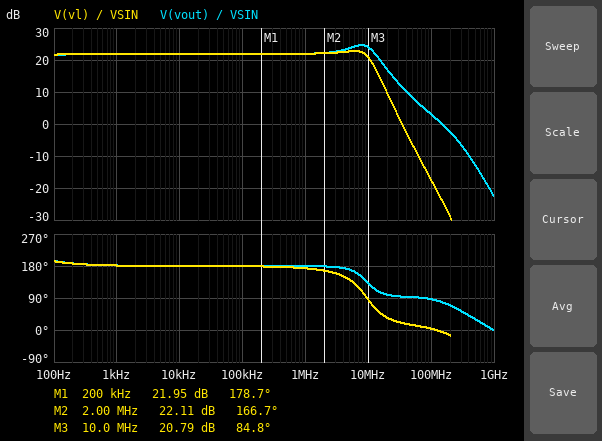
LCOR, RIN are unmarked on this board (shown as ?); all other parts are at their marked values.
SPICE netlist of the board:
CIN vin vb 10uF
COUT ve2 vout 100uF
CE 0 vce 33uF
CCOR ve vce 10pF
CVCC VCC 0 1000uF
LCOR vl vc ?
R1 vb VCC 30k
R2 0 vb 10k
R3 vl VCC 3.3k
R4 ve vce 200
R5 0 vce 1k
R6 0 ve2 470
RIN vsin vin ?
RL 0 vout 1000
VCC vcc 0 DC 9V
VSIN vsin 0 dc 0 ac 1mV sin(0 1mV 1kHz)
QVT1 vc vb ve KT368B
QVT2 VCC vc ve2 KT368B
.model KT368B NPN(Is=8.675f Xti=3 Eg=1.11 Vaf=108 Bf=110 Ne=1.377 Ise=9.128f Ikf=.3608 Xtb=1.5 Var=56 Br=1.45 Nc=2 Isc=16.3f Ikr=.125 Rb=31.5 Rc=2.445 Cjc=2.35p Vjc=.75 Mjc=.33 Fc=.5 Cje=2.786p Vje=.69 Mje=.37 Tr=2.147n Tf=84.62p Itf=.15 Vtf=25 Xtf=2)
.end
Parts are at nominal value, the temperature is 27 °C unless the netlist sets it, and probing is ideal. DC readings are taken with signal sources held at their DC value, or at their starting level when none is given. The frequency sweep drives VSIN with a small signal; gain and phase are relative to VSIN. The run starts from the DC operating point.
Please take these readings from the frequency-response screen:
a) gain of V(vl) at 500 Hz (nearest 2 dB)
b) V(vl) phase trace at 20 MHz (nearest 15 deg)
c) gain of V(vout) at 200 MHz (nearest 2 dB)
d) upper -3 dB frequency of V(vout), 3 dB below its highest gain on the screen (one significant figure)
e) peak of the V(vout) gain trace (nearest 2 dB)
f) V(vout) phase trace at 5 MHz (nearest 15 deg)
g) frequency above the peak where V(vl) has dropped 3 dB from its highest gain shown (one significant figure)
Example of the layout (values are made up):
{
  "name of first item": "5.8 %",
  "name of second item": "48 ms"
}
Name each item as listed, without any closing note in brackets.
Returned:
{
  "gain of V(vl) at 500 Hz": "22 dB",
  "V(vl) phase trace at 20 MHz": "30 deg",
  "gain of V(vout) at 200 MHz": "-2 dB",
  "upper -3 dB frequency of V(vout), 3 dB below its highest gain on the screen": "10 MHz",
  "peak of the V(vout) gain trace": "24 dB",
  "V(vout) phase trace at 5 MHz": "165 deg",
  "frequency above the peak where V(vl) has dropped 3 dB from its highest gain shown": "10 MHz"
}
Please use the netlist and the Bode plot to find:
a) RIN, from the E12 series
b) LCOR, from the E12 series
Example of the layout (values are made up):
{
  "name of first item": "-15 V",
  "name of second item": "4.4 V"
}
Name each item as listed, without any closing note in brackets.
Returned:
{
  "RIN, from the E12 series": "390 Ω",
  "LCOR, from the E12 series": "56 µH"
}
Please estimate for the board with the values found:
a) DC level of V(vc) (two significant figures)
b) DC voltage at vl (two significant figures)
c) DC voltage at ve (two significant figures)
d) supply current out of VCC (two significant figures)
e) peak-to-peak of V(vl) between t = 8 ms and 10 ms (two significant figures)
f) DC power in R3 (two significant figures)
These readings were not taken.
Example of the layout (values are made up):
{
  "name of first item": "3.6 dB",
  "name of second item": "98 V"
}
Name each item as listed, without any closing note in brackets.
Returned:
{
  "DC level of V(vc)": "4.7 V",
  "DC voltage at vl": "4.7 V",
  "DC voltage at ve": "1.5 V",
  "supply current out of VCC": "9.9 mA",
  "peak-to-peak of V(vl) between t = 8 ms and 10 ms": "25 mV",
  "DC power in R3": "5.7 mW"
}
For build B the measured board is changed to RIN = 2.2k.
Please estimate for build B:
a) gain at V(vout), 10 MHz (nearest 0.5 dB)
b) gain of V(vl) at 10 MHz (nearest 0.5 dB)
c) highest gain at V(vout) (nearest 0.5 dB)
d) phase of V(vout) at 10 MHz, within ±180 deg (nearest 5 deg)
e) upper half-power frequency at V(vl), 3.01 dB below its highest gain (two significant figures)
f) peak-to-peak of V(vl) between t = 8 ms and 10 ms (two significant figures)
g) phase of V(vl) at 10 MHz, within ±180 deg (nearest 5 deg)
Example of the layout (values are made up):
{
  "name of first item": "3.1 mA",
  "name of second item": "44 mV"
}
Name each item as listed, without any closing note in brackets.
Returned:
{
  "gain at V(vout), 10 MHz": "12.5 dB",
  "gain of V(vl) at 10 MHz": "9.5 dB",
  "highest gain at V(vout)": "19.5 dB",
  "phase of V(vout) at 10 MHz, within ±180 deg": "105 deg",
  "upper half-power frequency at V(vl), 3.01 dB below its highest gain": "5.0 MHz",
  "peak-to-peak of V(vl) between t = 8 ms and 10 ms": "19 mV",
  "phase of V(vl) at 10 MHz, within ±180 deg": "55 deg"
}
